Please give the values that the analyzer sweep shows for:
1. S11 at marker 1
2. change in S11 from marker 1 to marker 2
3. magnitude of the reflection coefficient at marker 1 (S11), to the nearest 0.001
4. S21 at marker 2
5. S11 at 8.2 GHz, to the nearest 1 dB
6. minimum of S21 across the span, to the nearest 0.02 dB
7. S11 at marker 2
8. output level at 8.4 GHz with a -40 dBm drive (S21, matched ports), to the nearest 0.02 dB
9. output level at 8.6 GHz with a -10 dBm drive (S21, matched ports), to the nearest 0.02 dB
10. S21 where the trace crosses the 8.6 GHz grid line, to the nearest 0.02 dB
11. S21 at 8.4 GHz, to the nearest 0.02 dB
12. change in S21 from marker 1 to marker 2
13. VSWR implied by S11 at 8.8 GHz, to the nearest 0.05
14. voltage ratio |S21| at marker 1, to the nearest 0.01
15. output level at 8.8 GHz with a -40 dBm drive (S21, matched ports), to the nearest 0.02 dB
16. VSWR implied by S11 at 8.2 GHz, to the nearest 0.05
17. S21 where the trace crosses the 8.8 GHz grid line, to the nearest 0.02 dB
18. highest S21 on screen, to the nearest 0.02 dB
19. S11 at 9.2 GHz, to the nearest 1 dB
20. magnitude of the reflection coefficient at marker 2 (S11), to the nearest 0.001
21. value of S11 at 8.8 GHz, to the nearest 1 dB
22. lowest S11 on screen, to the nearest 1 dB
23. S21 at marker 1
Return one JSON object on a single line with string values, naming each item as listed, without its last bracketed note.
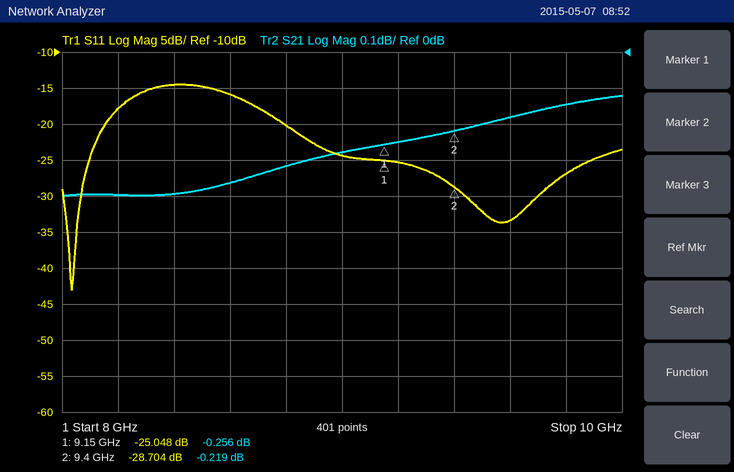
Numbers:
{"S11 at marker 1": "-25.048 dB", "change in S11 from marker 1 to marker 2": "-3.656 dB", "magnitude of the reflection coefficient at marker 1 (S11), to the nearest 0.001": "0.056", "S21 at marker 2": "-0.219 dB", "S11 at 8.2 GHz, to the nearest 1 dB": "-18 dB", "minimum of S21 across the span, to the nearest 0.02 dB": "-0.40 dB", "S11 at marker 2": "-28.704 dB", "output level at 8.4 GHz with a -40 dBm drive (S21, matched ports), to the nearest 0.02 dB": "-40.40 dBm", "output level at 8.6 GHz with a -10 dBm drive (S21, matched ports), to the nearest 0.02 dB": "-10.36 dBm", "S21 where the trace crosses the 8.6 GHz grid line, to the nearest 0.02 dB": "-0.36 dB", "S21 at 8.4 GHz, to the nearest 0.02 dB": "-0.40 dB", "change in S21 from marker 1 to marker 2": "0.037 dB", "VSWR implied by S11 at 8.8 GHz, to the nearest 0.05": "1.20", "voltage ratio |S21| at marker 1, to the nearest 0.01": "0.97", "output level at 8.8 GHz with a -40 dBm drive (S21, matched ports), to the nearest 0.02 dB": "-40.32 dBm", "VSWR implied by S11 at 8.2 GHz, to the nearest 0.05": "1.30", "S21 where the trace crosses the 8.8 GHz grid line, to the nearest 0.02 dB": "-0.32 dB", "highest S21 on screen, to the nearest 0.02 dB": "-0.12 dB", "S11 at 9.2 GHz, to the nearest 1 dB": "-25 dB", "magnitude of the reflection coefficient at marker 2 (S11), to the nearest 0.001": "0.037", "value of S11 at 8.8 GHz, to the nearest 1 dB": "-20 dB", "lowest S11 on screen, to the nearest 1 dB": "-43 dB", "S21 at marker 1": "-0.256 dB"}
